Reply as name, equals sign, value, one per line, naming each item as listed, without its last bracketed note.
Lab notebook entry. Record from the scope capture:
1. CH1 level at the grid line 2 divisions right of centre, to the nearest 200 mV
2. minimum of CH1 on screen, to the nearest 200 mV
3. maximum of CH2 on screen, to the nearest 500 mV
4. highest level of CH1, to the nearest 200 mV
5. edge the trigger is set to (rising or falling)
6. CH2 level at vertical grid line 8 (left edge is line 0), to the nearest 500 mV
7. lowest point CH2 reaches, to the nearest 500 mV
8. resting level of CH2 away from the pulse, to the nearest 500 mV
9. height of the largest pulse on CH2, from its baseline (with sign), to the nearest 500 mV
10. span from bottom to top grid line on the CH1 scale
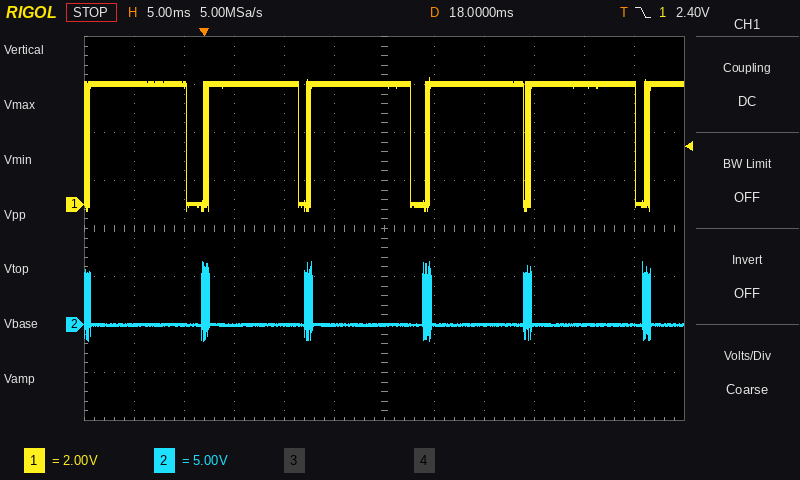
CH1 level at the grid line 2 divisions right of centre, to the nearest 200 mV = 5.0 V
minimum of CH1 on screen, to the nearest 200 mV = -200 mV
maximum of CH2 on screen, to the nearest 500 mV = 6.5 V
highest level of CH1, to the nearest 200 mV = 5.2 V
edge the trigger is set to = falling
CH2 level at vertical grid line 8 (left edge is line 0), to the nearest 500 mV = 0.0 V
lowest point CH2 reaches, to the nearest 500 mV = -1.5 V
resting level of CH2 away from the pulse, to the nearest 500 mV = 0.0 V
height of the largest pulse on CH2, from its baseline (with sign), to the nearest 500 mV = +6.5 V
span from bottom to top grid line on the CH1 scale = 16 V
